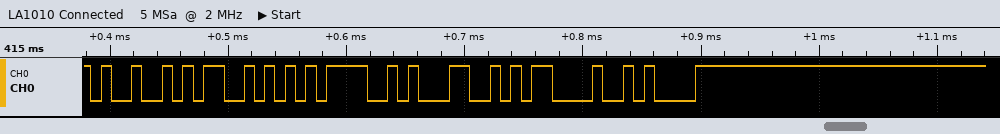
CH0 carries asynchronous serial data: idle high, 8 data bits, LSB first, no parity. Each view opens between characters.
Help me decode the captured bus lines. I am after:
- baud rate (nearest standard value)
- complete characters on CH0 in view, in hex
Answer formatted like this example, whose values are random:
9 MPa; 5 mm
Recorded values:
115200 baud; 49, 53, 3D, 31, 0D, 0A
